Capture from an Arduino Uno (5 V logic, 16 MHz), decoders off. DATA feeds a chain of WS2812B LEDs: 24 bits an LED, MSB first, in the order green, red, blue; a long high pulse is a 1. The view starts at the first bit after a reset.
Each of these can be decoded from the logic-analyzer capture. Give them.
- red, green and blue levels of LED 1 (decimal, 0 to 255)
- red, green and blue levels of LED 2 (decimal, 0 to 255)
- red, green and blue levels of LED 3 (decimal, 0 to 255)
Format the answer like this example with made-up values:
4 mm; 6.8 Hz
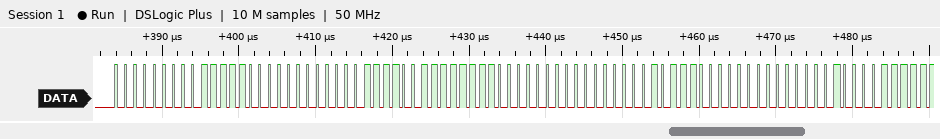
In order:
124, 0, 0; 255, 60, 0; 184, 0, 0
